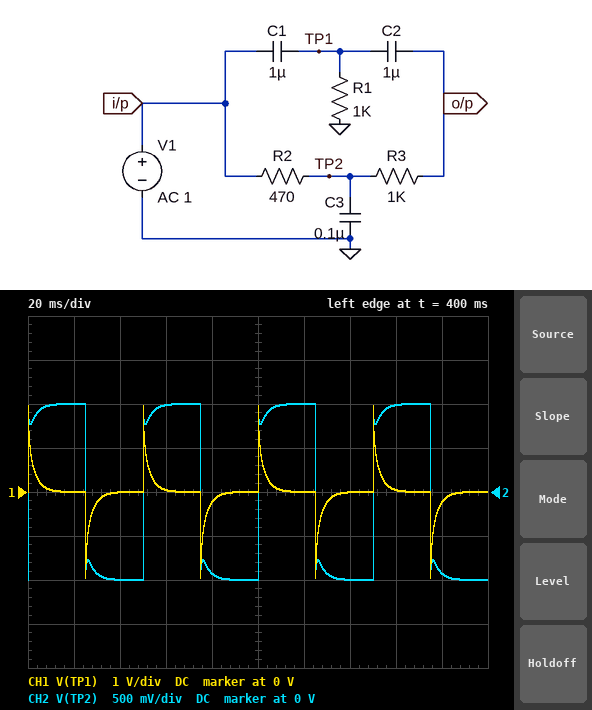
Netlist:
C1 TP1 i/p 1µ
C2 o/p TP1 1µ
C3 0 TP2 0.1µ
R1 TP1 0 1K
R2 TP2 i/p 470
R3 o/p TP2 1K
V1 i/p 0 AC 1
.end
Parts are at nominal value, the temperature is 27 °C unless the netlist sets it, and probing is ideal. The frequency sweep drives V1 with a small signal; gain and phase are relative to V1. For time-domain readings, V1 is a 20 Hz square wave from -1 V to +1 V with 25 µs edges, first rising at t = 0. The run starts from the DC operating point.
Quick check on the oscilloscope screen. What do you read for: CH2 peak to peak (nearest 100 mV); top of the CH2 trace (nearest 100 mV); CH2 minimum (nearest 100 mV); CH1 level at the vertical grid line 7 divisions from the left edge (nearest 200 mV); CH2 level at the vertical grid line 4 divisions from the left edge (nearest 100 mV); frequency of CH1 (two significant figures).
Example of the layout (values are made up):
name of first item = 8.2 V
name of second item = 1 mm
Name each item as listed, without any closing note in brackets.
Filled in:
CH2 peak to peak = 2.0 V
top of the CH2 trace = 1.0 V
CH2 minimum = -1.0 V
CH1 level at the vertical grid line 7 divisions from the left edge = 0 V
CH2 level at the vertical grid line 4 divisions from the left edge = -900 mV
frequency of CH1 = 20 Hz
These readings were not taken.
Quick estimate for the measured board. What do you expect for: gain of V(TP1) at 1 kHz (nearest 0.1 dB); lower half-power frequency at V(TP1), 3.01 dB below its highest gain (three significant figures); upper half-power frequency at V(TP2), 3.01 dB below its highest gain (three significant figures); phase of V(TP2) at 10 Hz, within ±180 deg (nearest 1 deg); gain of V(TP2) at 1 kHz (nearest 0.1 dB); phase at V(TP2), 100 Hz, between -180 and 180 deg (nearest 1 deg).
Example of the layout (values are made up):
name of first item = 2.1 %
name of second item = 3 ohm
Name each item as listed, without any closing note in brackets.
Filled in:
gain of V(TP1) at 1 kHz = -0.5 dB
lower half-power frequency at V(TP1), 3.01 dB below its highest gain = 164 Hz
upper half-power frequency at V(TP2), 3.01 dB below its highest gain = 4.86 kHz
phase of V(TP2) at 10 Hz, within ±180 deg = -2 deg
gain of V(TP2) at 1 kHz = -0.5 dB
phase at V(TP2), 100 Hz, between -180 and 180 deg = -3 deg
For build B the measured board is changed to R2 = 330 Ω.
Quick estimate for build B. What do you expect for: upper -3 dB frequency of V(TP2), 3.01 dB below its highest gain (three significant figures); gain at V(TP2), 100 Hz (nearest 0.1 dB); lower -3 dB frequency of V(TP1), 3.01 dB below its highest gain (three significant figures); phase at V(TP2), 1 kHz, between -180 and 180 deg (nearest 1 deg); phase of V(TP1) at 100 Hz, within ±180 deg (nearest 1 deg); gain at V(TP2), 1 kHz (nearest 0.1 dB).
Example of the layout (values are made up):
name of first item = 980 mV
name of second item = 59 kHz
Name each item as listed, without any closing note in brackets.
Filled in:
upper -3 dB frequency of V(TP2), 3.01 dB below its highest gain = 6.33 kHz
gain at V(TP2), 100 Hz = -0.9 dB
lower -3 dB frequency of V(TP1), 3.01 dB below its highest gain = 154 Hz
phase at V(TP2), 1 kHz, between -180 and 180 deg = -7 deg
phase of V(TP1) at 100 Hz, within ±180 deg = 35 deg
gain at V(TP2), 1 kHz = -0.3 dB
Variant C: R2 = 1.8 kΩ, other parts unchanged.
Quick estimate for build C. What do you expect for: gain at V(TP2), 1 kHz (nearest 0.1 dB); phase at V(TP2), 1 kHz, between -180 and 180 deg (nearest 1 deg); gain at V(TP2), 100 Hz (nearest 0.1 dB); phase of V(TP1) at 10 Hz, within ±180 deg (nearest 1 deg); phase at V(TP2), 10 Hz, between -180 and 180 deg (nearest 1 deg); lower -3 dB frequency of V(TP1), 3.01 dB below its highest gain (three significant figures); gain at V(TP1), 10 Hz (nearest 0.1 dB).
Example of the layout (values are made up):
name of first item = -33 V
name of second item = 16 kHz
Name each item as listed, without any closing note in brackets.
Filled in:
gain at V(TP2), 1 kHz = -1.5 dB
phase at V(TP2), 1 kHz, between -180 and 180 deg = -16 deg
gain at V(TP2), 100 Hz = -4.3 dB
phase of V(TP1) at 10 Hz, within ±180 deg = 78 deg
phase at V(TP2), 10 Hz, between -180 and 180 deg = -7 deg
lower -3 dB frequency of V(TP1), 3.01 dB below its highest gain = 197 Hz
gain at V(TP1), 10 Hz = -18.3 dB
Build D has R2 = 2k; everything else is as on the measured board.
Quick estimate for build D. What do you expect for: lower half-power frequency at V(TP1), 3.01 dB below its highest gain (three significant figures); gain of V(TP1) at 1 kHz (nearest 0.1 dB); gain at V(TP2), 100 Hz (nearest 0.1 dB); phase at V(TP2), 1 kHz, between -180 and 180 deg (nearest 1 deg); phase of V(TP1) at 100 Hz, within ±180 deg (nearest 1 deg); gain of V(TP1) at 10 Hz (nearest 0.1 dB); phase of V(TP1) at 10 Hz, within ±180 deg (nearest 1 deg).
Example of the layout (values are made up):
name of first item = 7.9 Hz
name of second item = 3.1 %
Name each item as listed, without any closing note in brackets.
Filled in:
lower half-power frequency at V(TP1), 3.01 dB below its highest gain = 198 Hz
gain of V(TP1) at 1 kHz = -0.7 dB
gain at V(TP2), 100 Hz = -4.7 dB
phase at V(TP2), 1 kHz, between -180 and 180 deg = -16 deg
phase of V(TP1) at 100 Hz, within ±180 deg = 39 deg
gain of V(TP1) at 10 Hz = -18.3 dB
phase of V(TP1) at 10 Hz, within ±180 deg = 77 deg
